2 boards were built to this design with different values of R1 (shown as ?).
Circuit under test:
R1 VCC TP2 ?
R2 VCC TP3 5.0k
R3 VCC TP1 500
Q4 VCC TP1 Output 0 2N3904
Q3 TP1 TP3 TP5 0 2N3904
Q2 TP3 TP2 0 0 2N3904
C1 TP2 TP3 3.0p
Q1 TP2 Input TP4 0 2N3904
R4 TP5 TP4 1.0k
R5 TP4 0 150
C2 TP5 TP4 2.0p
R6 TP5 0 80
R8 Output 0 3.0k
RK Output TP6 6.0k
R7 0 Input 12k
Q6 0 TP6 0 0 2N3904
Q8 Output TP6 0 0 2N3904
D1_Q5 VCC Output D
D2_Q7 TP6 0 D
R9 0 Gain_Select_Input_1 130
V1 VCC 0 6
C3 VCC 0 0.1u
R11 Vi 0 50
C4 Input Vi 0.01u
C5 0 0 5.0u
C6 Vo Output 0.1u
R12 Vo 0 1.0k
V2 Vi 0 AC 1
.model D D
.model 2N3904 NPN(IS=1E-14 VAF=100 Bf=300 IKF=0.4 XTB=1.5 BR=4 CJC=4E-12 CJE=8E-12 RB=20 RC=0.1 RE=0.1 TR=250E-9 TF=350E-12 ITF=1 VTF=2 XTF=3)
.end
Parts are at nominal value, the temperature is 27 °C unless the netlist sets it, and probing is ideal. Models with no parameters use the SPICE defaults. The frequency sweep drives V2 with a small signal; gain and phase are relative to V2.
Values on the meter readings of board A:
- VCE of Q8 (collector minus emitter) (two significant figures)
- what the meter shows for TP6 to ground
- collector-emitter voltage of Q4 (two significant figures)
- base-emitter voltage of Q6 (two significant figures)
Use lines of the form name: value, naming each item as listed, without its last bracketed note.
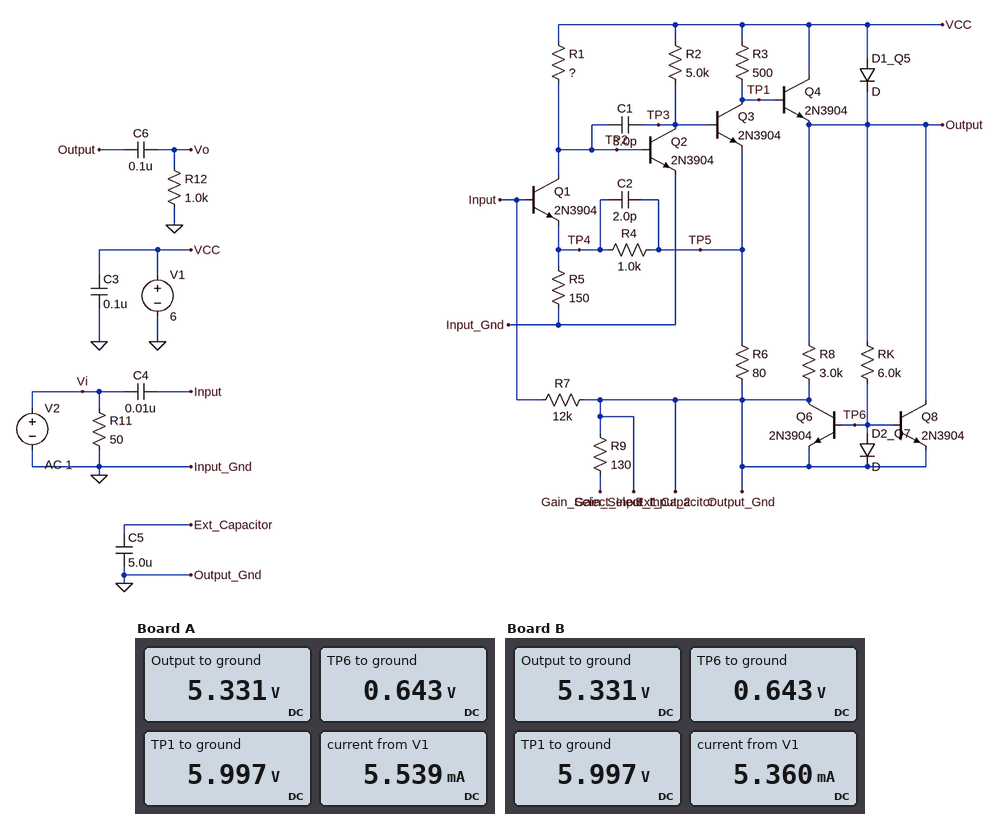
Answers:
VCE of Q8 (collector minus emitter): 5.3 V
what the meter shows for TP6 to ground: 0.643 V
collector-emitter voltage of Q4: 670 mV
base-emitter voltage of Q6: 640 mV
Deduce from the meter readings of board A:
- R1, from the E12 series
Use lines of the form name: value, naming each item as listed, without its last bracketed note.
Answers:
R1, from the E12 series: 4.7 kΩ
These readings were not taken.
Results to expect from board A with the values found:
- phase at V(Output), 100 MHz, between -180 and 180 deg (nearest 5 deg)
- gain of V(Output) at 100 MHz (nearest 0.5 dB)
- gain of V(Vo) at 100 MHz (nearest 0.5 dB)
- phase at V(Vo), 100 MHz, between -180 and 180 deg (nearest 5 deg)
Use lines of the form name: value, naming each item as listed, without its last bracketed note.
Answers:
phase at V(Output), 100 MHz, between -180 and 180 deg: 125 deg
gain of V(Output) at 100 MHz: -69.0 dB
gain of V(Vo) at 100 MHz: -69.0 dB
phase at V(Vo), 100 MHz, between -180 and 180 deg: 125 deg
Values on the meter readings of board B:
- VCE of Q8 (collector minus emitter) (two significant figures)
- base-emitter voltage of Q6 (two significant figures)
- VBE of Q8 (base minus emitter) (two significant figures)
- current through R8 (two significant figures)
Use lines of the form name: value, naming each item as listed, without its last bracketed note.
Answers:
VCE of Q8 (collector minus emitter): 5.3 V
base-emitter voltage of Q6: 640 mV
VBE of Q8 (base minus emitter): 640 mV
current through R8: 1.8 mA
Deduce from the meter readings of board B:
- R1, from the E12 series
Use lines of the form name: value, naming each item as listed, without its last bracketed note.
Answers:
R1, from the E12 series: 5.6 kΩ
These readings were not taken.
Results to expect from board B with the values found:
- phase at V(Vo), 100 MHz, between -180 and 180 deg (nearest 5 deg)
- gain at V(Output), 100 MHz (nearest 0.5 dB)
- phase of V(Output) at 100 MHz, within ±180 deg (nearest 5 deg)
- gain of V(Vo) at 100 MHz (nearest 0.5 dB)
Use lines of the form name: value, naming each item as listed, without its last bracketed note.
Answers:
phase at V(Vo), 100 MHz, between -180 and 180 deg: 120 deg
gain at V(Output), 100 MHz: -68.5 dB
phase of V(Output) at 100 MHz, within ±180 deg: 120 deg
gain of V(Vo) at 100 MHz: -68.5 dB
